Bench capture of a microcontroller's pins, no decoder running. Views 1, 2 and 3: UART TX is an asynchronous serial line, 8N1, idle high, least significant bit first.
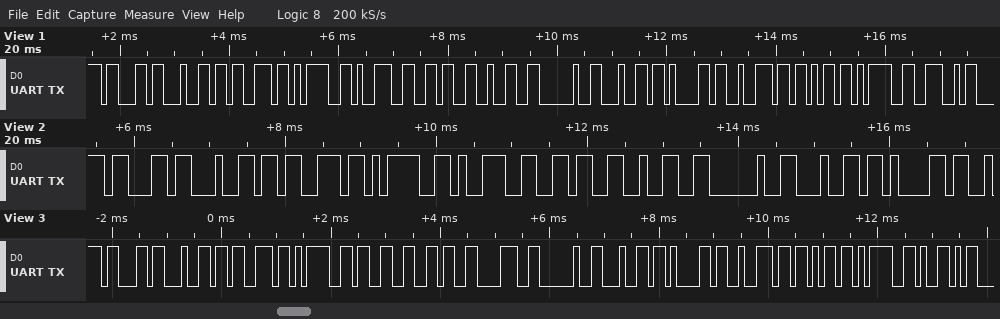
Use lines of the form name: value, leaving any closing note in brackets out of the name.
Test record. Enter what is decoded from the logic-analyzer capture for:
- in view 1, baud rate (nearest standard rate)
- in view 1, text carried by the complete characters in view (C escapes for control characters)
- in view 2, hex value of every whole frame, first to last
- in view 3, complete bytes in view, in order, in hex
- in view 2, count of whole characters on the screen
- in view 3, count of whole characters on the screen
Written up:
in view 1, baud rate: 9600 baud
in view 1, text carried by the complete characters in view: "cds=962 dark=N"
in view 2, hex value of every whole frame, first to last: 0x63 0x64 0x73 0x3D 0x39 0x36 0x32 0x20 0x64 0x61
in view 3, complete bytes in view, in order, in hex: 63 64 73 3D 33 36 38 20 64 61 72 6B 3D 59
in view 2, count of whole characters on the screen: 10
in view 3, count of whole characters on the screen: 14
